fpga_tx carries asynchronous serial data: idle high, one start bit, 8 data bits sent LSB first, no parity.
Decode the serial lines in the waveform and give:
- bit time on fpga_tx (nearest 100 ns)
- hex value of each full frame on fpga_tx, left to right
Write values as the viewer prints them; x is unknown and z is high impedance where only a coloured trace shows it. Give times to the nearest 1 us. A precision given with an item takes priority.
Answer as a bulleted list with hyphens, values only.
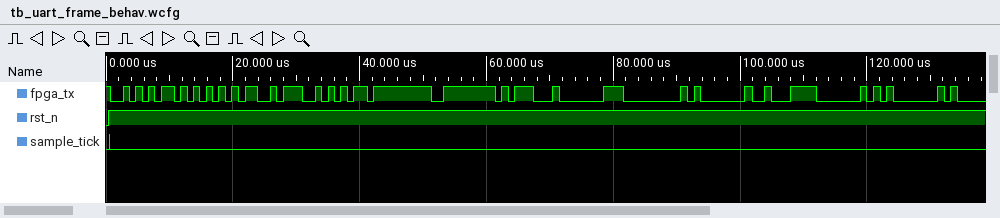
- 1000 ns
- AA, 55, D3, AA, FF, FE, 1D, C0, 00, 01, E2, 40, 01
